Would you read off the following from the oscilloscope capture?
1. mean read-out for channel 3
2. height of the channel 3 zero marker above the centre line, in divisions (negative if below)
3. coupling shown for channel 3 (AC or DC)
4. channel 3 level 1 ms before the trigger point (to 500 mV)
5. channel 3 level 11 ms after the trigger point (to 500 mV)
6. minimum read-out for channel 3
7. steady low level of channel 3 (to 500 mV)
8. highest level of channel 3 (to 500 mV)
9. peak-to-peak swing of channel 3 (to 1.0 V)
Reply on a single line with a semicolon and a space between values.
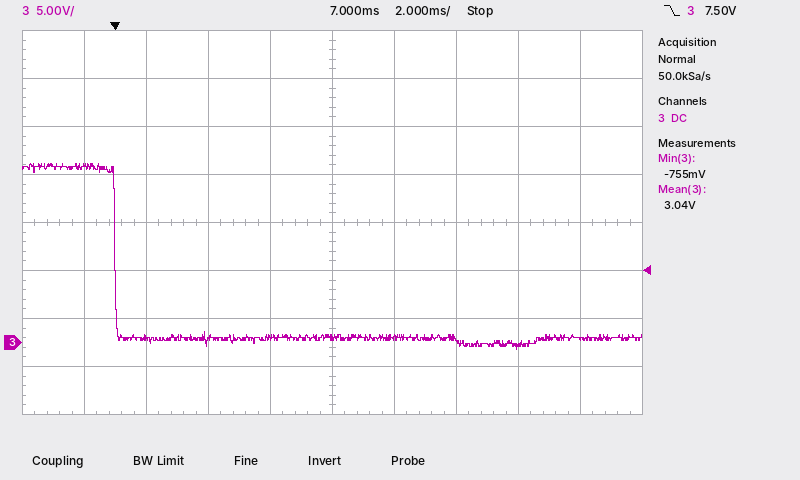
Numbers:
3.04 V; -2.5 div; DC; 18.5 V; 500 mV; -755 mV; 500 mV; 18.5 V; 19.0 V
